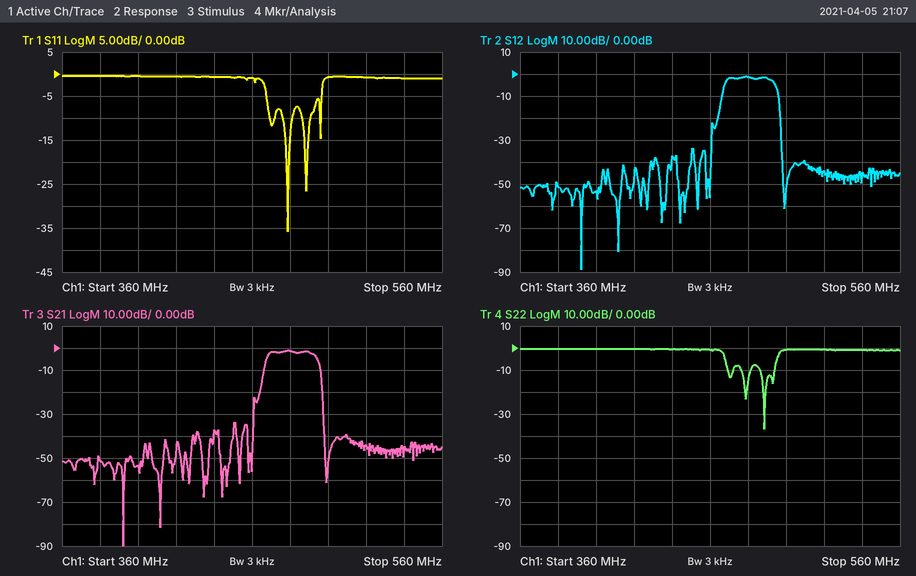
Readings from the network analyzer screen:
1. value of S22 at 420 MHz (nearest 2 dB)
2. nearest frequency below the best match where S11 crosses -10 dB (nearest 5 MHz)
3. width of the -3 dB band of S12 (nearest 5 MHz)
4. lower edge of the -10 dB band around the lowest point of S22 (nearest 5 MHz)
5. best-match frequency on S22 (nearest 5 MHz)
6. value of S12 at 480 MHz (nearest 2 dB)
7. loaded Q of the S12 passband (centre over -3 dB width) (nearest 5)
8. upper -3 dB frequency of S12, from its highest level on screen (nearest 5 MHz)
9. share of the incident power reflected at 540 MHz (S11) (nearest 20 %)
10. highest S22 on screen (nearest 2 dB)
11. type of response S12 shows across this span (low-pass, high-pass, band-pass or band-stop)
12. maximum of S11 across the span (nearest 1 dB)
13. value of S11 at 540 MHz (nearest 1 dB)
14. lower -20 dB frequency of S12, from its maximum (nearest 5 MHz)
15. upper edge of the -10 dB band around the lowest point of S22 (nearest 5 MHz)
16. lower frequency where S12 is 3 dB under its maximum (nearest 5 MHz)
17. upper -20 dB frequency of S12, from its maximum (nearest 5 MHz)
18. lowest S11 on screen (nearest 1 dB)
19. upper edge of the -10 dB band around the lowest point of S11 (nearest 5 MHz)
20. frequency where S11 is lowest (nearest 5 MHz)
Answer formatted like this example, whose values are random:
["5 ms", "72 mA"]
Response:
["0 dB", "475 MHz", "25 MHz", "485 MHz", "490 MHz", "-2 dB", "20", "495 MHz", "80 %", "0 dB", "band-pass", "0 dB", "-1 dB", "465 MHz", "495 MHz", "470 MHz", "495 MHz", "-36 dB", "480 MHz", "480 MHz"]
